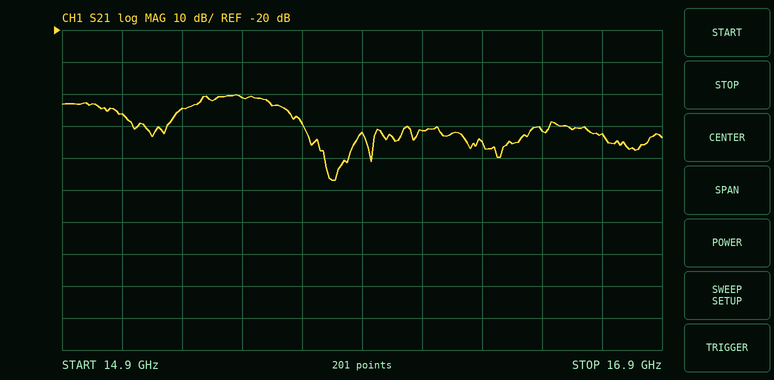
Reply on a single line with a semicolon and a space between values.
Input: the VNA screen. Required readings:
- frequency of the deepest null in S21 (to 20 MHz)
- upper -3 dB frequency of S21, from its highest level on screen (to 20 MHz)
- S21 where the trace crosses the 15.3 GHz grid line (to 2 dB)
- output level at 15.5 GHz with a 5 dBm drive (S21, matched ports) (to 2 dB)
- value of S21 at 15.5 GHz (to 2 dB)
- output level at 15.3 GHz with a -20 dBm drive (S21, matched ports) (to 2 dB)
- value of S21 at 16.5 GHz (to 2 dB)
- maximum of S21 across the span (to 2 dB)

15.80 GHz; 15.60 GHz; -44 dB; -36 dBm; -42 dB; -64 dBm; -52 dB; -40 dB
